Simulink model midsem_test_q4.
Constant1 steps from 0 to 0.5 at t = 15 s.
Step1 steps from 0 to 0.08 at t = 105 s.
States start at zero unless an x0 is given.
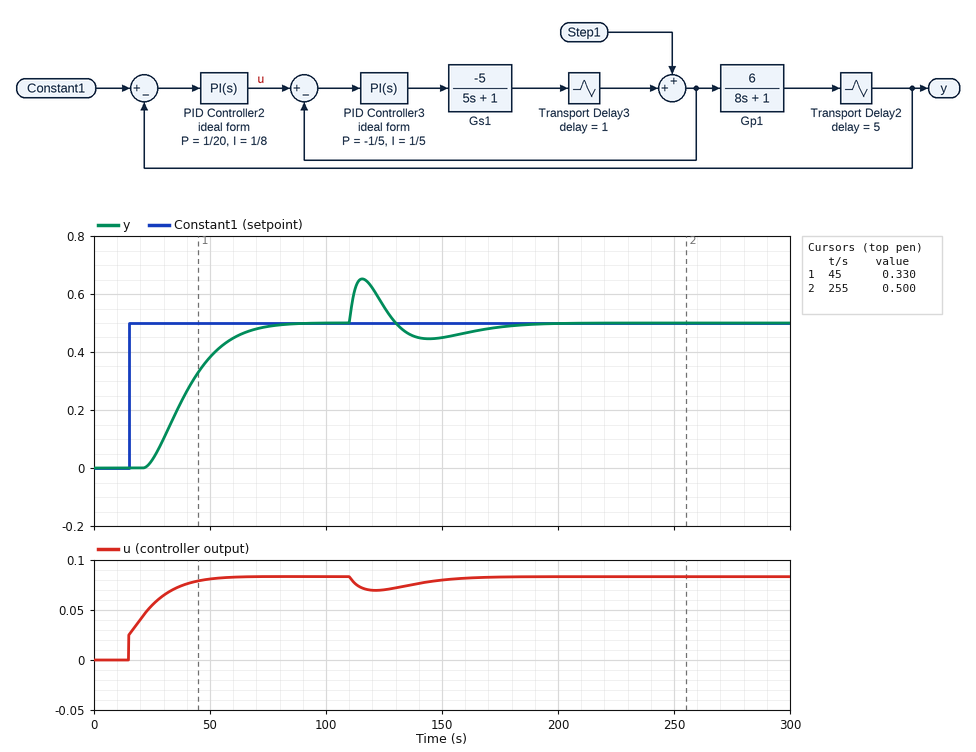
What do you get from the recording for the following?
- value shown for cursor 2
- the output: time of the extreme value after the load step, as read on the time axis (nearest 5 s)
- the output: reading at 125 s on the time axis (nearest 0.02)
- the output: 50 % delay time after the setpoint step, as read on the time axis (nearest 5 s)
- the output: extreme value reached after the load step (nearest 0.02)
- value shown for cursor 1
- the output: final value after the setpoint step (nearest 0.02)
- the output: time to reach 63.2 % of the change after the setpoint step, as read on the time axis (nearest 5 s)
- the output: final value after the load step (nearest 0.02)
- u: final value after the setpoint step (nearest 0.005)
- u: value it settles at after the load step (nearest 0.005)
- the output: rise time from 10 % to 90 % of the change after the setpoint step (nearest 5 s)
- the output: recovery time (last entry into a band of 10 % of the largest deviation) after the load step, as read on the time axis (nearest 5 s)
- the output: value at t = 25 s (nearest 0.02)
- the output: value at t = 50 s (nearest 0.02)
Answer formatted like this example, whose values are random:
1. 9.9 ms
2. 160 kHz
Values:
1. 0.500
2. 115 s
3. 0.56
4. 40 s
5. 0.66
6. 0.330
7. 0.50
8. 45 s
9. 0.50
10. 0.085
11. 0.085
12. 35 s
13. 175 s
14. 0.02
15. 0.38
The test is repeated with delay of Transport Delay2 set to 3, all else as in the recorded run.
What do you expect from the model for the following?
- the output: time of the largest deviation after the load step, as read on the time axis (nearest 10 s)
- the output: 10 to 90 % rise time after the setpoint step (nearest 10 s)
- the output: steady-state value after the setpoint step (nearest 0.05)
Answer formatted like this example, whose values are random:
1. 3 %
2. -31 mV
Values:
1. 110 s
2. 40 s
3. 0.50
